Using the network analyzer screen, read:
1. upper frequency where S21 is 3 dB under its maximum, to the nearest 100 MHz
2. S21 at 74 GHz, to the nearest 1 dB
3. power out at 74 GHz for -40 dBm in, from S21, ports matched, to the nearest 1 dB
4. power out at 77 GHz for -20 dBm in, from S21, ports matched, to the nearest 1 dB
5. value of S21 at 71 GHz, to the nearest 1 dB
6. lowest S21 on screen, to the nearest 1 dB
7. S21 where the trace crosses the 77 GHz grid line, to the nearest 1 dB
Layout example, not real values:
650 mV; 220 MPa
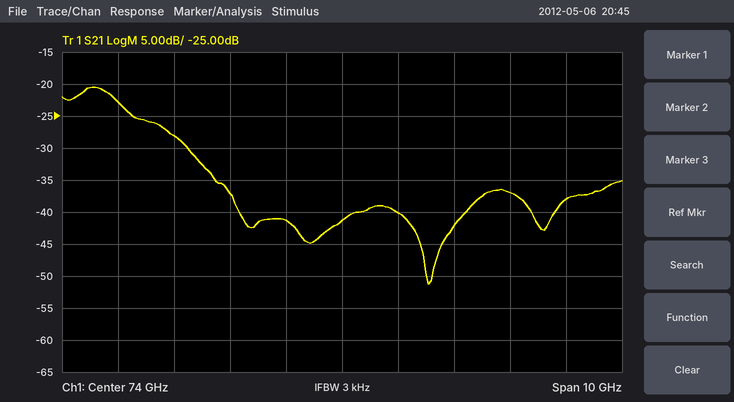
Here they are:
70.1 GHz; -41 dB; -81 dBm; -57 dBm; -28 dB; -51 dB; -37 dB
